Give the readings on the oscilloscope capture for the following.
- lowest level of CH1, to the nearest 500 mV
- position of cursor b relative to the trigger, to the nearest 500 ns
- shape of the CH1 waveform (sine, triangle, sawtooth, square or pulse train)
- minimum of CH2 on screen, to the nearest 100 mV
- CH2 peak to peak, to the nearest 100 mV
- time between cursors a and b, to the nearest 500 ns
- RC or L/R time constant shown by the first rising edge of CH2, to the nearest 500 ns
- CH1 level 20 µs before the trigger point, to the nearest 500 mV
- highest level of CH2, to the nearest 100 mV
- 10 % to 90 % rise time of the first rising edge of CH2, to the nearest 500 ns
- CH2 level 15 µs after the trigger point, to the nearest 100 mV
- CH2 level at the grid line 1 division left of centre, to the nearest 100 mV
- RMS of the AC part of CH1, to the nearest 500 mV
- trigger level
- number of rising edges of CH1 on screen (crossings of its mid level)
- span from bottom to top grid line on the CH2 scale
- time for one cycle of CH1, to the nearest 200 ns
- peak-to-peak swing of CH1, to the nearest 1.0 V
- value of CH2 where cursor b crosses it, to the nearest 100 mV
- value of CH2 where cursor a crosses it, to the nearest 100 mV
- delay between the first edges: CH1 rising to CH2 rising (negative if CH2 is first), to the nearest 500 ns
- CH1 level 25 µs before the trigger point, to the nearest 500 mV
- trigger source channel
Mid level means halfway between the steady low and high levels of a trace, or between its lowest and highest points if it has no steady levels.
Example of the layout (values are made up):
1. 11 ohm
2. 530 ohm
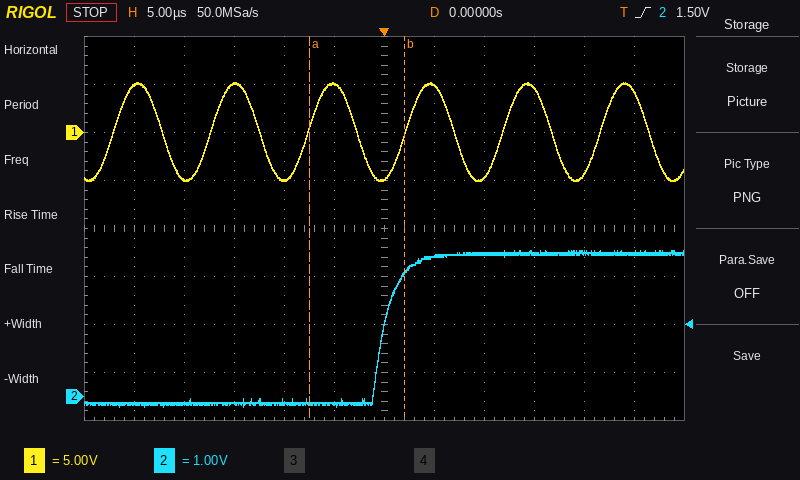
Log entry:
1. -5.0 V
2. +2.0 µs
3. sine
4. -200 mV
5. 3.2 V
6. 9.5 µs
7. 1.5 µs
8. -5.0 V
9. 3.0 V
10. 3.5 µs
11. 3.0 V
12. -200 mV
13. 3.5 V
14. 1.50 V
15. 6
16. 8 V
17. 9.8 µs
18. 10.0 V
19. 2.6 V
20. -100 mV
21. +27.0 µs
22. 5.0 V
23. CH2
